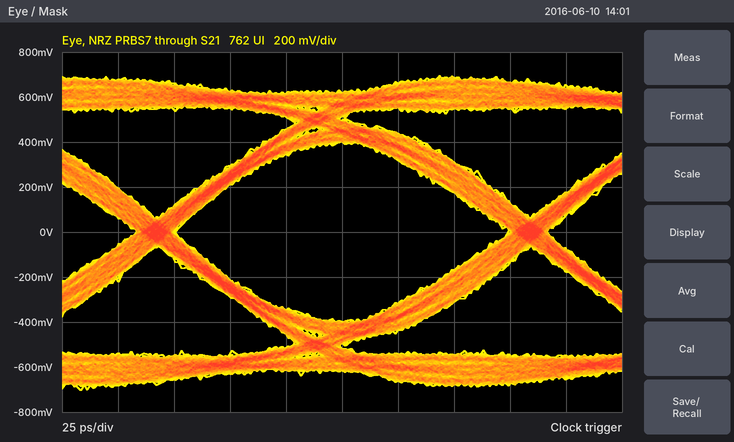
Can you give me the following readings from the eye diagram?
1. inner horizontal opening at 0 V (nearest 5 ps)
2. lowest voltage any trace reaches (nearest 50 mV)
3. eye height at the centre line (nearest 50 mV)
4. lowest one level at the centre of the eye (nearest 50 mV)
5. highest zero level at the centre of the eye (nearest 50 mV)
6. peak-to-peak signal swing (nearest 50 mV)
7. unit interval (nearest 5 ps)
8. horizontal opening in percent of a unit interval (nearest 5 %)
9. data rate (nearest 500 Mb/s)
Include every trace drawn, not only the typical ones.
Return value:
150 ps
-700 mV
800 mV
400 mV
-400 mV
1.40 V
165 ps
90 %
6.0 Gb/s
